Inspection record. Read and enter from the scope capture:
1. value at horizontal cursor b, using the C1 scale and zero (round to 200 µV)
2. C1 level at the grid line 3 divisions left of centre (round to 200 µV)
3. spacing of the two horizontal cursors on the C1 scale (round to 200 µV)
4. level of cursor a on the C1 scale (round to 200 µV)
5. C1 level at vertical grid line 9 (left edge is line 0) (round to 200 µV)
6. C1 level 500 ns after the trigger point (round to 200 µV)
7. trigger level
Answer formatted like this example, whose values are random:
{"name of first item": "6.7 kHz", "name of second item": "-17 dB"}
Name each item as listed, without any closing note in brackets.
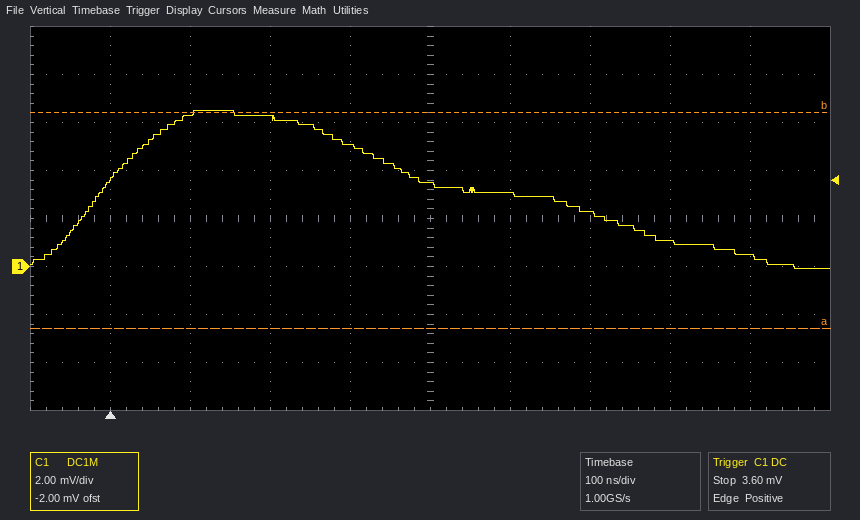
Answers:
{"value at horizontal cursor b, using the C1 scale and zero": "6.4 mV", "C1 level at the grid line 3 divisions left of centre": "6.4 mV", "spacing of the two horizontal cursors on the C1 scale": "9.0 mV", "level of cursor a on the C1 scale": "-2.6 mV", "C1 level at vertical grid line 9 (left edge is line 0)": "400 µV", "C1 level 500 ns after the trigger point": "3.0 mV", "trigger level": "3.60 mV"}
